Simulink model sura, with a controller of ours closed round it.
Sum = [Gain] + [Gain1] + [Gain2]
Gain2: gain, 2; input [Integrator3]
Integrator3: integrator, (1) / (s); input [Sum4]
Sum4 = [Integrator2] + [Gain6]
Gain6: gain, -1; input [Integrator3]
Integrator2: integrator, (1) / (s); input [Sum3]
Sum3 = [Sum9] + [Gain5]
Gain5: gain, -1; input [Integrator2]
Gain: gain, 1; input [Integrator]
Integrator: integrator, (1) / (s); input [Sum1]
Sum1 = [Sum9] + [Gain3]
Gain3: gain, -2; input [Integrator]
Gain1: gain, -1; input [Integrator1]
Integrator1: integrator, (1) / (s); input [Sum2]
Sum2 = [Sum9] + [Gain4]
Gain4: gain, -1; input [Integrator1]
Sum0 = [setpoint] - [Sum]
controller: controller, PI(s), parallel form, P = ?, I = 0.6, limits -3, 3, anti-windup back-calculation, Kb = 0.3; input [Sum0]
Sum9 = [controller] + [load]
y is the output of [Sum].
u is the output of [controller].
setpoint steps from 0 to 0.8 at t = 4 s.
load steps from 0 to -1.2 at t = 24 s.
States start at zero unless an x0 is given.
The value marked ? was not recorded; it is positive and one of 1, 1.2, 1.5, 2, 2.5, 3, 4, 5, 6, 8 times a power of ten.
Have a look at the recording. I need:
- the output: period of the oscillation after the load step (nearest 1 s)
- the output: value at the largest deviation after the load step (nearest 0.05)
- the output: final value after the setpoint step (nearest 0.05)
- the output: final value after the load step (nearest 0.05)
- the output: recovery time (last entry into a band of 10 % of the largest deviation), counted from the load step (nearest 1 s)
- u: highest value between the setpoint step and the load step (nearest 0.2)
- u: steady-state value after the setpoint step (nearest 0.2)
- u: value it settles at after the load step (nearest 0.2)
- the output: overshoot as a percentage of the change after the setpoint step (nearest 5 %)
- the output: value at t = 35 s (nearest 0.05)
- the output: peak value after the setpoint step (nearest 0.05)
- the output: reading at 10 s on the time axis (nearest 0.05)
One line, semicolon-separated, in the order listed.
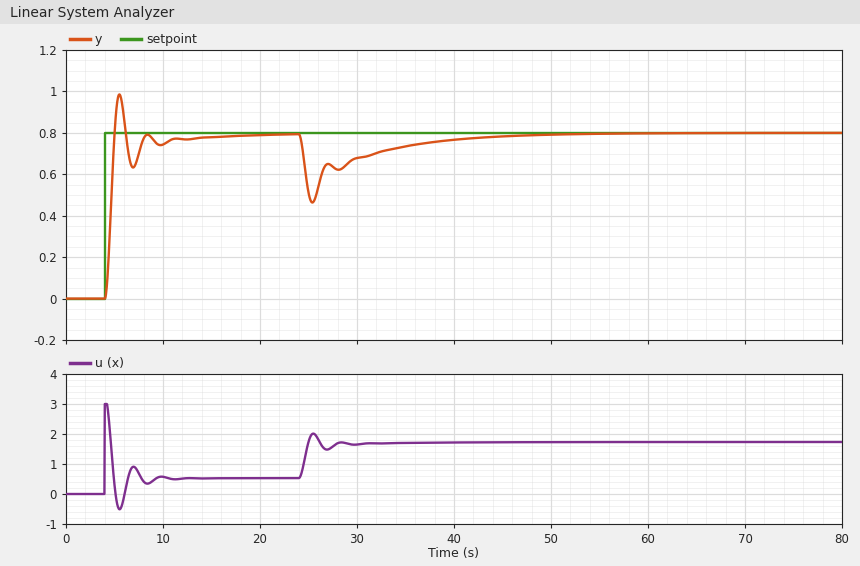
3 s; 0.45; 0.80; 0.80; 16 s; 3.0; 0.6; 1.8; 25 %; 0.75; 1.00; 0.75
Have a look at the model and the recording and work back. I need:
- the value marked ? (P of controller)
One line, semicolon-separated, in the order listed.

4
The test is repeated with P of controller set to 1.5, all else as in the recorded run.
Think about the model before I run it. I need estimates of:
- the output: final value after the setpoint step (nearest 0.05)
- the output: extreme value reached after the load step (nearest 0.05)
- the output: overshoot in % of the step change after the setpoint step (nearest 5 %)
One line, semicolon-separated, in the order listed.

0.80; 0.25; 10 %
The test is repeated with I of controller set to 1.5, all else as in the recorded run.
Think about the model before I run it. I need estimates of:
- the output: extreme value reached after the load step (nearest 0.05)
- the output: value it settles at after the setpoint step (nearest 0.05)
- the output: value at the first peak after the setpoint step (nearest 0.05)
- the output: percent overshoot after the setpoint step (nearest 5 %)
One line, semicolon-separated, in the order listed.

0.50; 0.80; 1.10; 35 %
